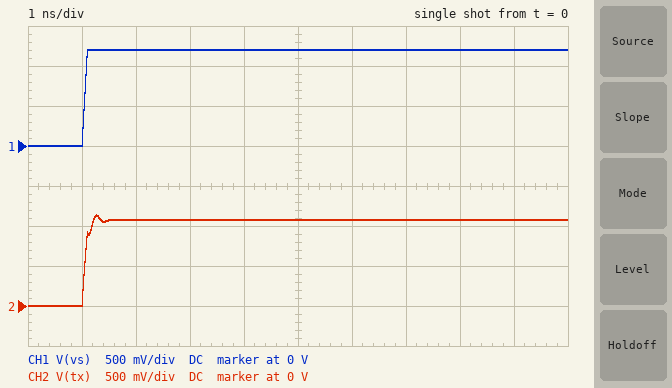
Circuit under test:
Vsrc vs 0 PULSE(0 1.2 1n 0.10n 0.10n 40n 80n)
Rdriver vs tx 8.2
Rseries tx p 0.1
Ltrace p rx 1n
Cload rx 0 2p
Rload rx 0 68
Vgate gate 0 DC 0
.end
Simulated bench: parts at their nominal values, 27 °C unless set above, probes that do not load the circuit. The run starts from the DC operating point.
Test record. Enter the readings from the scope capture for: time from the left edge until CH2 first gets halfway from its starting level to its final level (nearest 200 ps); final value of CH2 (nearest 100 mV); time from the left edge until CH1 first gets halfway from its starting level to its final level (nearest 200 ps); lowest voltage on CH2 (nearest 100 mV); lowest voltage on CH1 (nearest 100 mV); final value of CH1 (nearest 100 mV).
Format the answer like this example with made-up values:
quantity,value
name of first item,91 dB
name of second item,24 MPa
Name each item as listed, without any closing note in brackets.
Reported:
quantity,value
time from the left edge until CH2 first gets halfway from its starting level to its final level,1.0 ns
final value of CH2,1.1 V
time from the left edge until CH1 first gets halfway from its starting level to its final level,1.0 ns
lowest voltage on CH2,0 V
lowest voltage on CH1,0 V
final value of CH1,1.2 V
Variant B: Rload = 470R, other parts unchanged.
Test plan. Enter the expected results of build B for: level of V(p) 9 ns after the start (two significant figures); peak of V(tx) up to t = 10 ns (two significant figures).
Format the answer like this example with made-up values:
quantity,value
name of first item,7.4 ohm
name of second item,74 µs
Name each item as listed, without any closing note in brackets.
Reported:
quantity,value
level of V(p) 9 ns after the start,1.2 V
peak of V(tx) up to t = 10 ns,1.3 V
